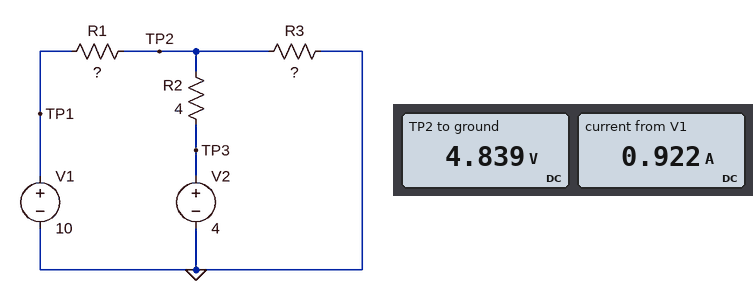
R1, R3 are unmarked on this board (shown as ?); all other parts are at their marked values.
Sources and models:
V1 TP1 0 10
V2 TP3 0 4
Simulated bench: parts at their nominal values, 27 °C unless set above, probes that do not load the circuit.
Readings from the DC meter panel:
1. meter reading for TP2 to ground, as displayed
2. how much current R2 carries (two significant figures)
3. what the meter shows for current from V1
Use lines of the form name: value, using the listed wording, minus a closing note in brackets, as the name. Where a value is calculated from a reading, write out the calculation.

meter reading for TP2 to ground, as displayed: 4.839 V
how much current R2 carries: (4.839 V - 4 V) / 4 Ω = 210 mA
what the meter shows for current from V1: 0.922 A
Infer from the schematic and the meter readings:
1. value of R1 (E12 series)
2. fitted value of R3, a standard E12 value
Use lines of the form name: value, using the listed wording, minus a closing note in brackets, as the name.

value of R1: 5.6 Ω
fitted value of R3, a standard E12 value: 6.8 Ω
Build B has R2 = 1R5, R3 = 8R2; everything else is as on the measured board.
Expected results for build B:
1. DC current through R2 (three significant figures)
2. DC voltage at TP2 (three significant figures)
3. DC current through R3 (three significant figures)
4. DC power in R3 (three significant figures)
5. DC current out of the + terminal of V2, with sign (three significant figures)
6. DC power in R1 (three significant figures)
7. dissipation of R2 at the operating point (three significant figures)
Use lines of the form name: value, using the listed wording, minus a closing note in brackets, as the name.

DC current through R2: 402 mA
DC voltage at TP2: 4.60 V
DC current through R3: 561 mA
DC power in R3: 2.58 W
DC current out of the + terminal of V2, with sign: -402 mA
DC power in R1: 5.20 W
dissipation of R2 at the operating point: 243 mW
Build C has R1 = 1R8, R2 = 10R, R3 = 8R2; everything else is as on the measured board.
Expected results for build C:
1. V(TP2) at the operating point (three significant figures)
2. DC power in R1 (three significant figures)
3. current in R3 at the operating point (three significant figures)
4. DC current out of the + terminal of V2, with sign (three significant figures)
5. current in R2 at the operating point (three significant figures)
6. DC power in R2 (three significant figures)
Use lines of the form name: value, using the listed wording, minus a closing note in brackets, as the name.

V(TP2) at the operating point: 7.66 V
DC power in R1: 3.04 W
current in R3 at the operating point: 934 mA
DC current out of the + terminal of V2, with sign: -366 mA
current in R2 at the operating point: 366 mA
DC power in R2: 1.34 W
